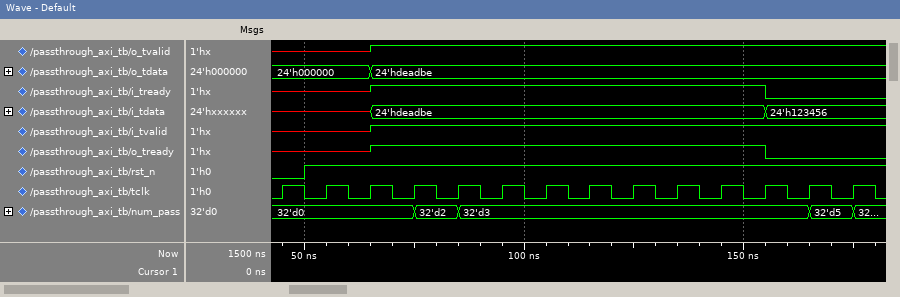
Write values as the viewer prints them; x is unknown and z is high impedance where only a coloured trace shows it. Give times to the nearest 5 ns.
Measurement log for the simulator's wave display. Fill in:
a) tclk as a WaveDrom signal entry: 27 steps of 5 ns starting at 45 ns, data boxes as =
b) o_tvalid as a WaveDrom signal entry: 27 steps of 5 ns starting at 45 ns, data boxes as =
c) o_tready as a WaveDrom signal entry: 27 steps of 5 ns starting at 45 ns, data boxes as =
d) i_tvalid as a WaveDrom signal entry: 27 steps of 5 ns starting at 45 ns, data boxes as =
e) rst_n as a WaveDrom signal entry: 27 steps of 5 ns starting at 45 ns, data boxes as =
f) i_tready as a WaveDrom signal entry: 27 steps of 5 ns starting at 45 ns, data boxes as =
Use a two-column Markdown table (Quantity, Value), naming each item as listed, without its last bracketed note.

| Quantity | Value |
|---|---|
| tclk as a WaveDrom signal entry: 27 steps of 5 ns starting at 45 ns, data boxes as = | {name: 'tclk', wave: '101010101010101010101010101'} |
| o_tvalid as a WaveDrom signal entry: 27 steps of 5 ns starting at 45 ns, data boxes as = | {name: 'o_tvalid', wave: 'x...1......................'} |
| o_tready as a WaveDrom signal entry: 27 steps of 5 ns starting at 45 ns, data boxes as = | {name: 'o_tready', wave: 'x...1.................0....'} |
| i_tvalid as a WaveDrom signal entry: 27 steps of 5 ns starting at 45 ns, data boxes as = | {name: 'i_tvalid', wave: 'x...1......................'} |
| rst_n as a WaveDrom signal entry: 27 steps of 5 ns starting at 45 ns, data boxes as = | {name: 'rst_n', wave: '01.........................'} |
| i_tready as a WaveDrom signal entry: 27 steps of 5 ns starting at 45 ns, data boxes as = | {name: 'i_tready', wave: 'x...1.................0....'} |
